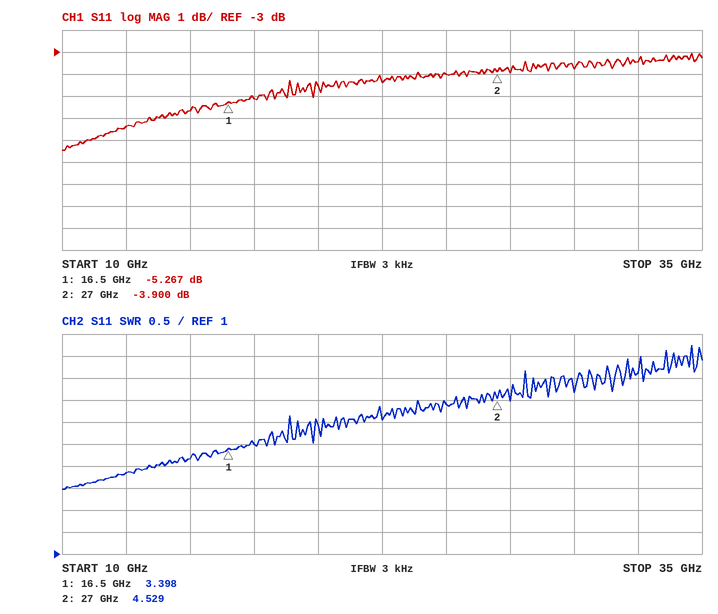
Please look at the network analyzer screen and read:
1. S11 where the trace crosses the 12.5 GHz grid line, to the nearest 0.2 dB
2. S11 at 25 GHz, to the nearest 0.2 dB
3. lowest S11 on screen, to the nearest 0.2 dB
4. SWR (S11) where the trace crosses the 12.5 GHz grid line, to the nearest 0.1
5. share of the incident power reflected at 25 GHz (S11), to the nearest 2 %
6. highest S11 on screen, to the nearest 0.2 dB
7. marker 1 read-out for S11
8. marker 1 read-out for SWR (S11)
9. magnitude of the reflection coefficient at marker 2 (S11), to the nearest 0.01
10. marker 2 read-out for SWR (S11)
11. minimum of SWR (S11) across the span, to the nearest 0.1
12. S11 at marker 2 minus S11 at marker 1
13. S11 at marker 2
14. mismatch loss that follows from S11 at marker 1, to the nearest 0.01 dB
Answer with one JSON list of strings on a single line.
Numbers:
["-6.4 dB", "-4.0 dB", "-7.4 dB", "2.8", "40 %", "-3.0 dB", "-5.267 dB", "3.398", "0.64", "4.529", "2.5", "1.367 dB", "-3.900 dB", "1.53 dB"]
